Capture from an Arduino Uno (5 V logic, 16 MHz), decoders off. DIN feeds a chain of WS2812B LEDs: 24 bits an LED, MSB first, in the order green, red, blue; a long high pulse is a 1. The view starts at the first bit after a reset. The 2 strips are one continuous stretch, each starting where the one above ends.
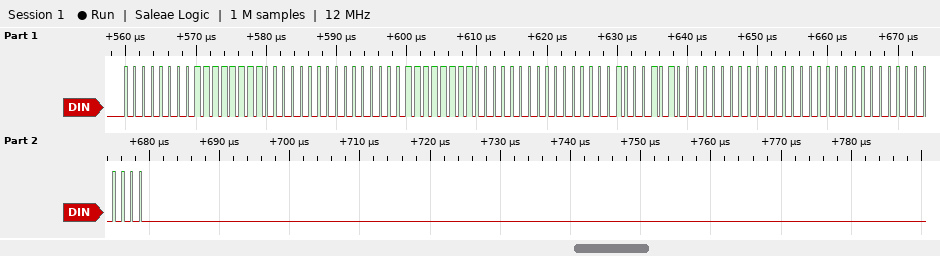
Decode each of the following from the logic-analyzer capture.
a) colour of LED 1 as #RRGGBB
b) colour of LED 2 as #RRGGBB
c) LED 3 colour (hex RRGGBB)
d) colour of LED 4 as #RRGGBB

#FF0000
#FF0000
#8A0000
#000000
